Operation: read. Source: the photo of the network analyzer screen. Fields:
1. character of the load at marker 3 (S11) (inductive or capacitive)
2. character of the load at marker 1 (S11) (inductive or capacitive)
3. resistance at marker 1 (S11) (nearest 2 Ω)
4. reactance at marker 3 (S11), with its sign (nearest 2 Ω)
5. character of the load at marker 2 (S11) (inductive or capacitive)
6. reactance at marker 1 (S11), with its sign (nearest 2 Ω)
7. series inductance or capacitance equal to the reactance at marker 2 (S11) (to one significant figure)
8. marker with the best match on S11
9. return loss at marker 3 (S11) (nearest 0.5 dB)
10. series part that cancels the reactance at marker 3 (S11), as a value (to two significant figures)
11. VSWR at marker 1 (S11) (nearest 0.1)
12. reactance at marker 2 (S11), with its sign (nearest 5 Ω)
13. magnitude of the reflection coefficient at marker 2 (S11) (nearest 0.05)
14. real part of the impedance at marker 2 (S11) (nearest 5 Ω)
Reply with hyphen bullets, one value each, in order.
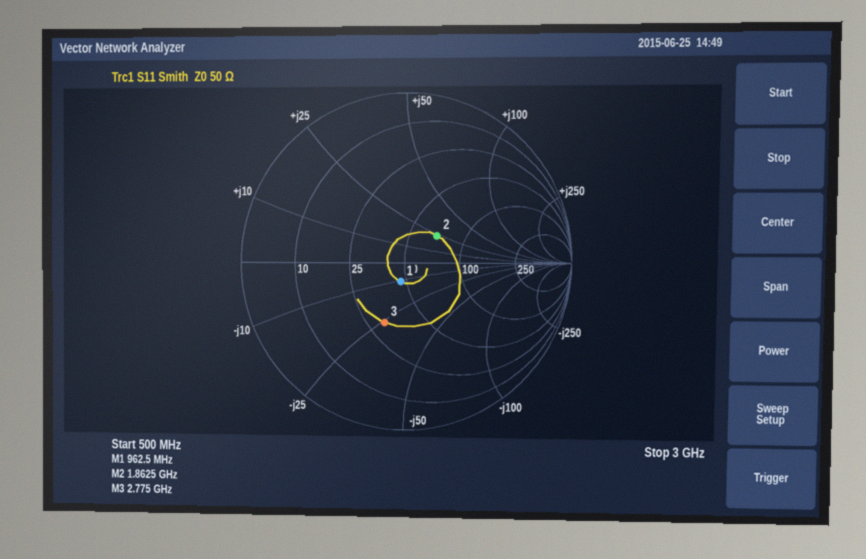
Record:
- capacitive
- capacitive
- 46 Ω
- -26 Ω
- inductive
- -10 Ω
- 2 nH
- marker 1
- 8.5 dB
- 1.5 nH
- 1.3
- +25 Ω
- 0.25
- 70 Ω
